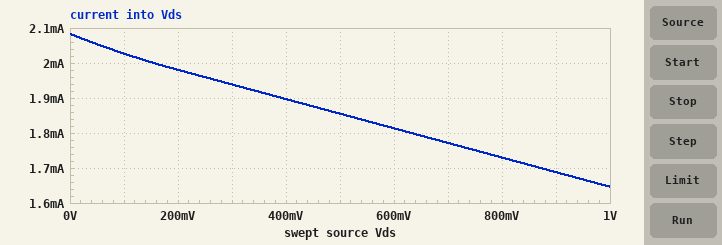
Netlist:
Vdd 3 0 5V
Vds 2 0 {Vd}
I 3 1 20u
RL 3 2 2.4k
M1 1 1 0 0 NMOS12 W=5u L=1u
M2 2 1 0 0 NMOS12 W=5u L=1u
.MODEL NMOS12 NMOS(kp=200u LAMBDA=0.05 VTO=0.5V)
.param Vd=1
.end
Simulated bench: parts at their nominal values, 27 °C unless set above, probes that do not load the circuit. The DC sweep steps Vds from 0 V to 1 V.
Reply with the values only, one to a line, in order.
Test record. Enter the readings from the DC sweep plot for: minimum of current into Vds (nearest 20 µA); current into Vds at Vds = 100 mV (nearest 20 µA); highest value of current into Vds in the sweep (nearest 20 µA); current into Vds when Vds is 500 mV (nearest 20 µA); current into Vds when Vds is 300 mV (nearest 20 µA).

1.64 mA
2.02 mA
2.08 mA
1.86 mA
1.94 mA
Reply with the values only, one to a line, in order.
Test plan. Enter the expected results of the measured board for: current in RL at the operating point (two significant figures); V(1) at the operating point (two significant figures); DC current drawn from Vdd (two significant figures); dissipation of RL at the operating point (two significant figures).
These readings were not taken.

1.7 mA
700 mV
1.7 mA
6.7 mW
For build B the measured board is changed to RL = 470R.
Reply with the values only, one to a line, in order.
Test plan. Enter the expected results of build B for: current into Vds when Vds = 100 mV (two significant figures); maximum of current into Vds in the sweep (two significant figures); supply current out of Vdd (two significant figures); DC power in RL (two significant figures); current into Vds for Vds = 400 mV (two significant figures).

10 mA
11 mA
8.5 mA
34 mW
9.8 mA
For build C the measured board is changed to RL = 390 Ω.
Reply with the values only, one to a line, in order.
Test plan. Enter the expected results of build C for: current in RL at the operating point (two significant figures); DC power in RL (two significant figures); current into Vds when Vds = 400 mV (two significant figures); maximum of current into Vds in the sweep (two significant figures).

10 mA
41 mW
12 mA
13 mA
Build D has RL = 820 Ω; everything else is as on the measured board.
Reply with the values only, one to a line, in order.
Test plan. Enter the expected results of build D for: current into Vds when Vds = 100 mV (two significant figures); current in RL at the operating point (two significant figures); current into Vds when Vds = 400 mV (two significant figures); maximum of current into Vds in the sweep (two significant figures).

6.0 mA
4.9 mA
5.6 mA
6.1 mA
